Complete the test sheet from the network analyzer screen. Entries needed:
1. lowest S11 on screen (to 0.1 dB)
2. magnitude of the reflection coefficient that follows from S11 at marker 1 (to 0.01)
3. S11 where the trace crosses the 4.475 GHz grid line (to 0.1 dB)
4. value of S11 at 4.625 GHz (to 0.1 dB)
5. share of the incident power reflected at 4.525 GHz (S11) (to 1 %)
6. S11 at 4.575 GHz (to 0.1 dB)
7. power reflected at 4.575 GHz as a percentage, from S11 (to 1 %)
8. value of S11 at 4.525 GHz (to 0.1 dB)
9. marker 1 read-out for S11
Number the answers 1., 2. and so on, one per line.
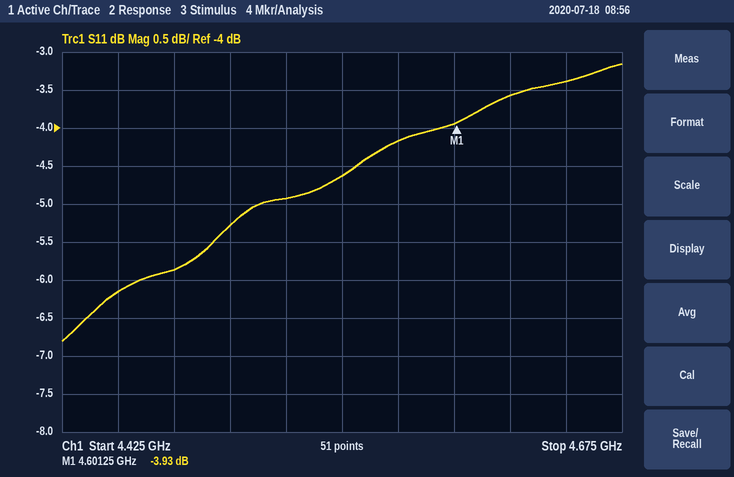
1. -6.8 dB
2. 0.64
3. -5.9 dB
4. -3.6 dB
5. 32 %
6. -4.2 dB
7. 38 %
8. -4.9 dB
9. -3.93 dB
